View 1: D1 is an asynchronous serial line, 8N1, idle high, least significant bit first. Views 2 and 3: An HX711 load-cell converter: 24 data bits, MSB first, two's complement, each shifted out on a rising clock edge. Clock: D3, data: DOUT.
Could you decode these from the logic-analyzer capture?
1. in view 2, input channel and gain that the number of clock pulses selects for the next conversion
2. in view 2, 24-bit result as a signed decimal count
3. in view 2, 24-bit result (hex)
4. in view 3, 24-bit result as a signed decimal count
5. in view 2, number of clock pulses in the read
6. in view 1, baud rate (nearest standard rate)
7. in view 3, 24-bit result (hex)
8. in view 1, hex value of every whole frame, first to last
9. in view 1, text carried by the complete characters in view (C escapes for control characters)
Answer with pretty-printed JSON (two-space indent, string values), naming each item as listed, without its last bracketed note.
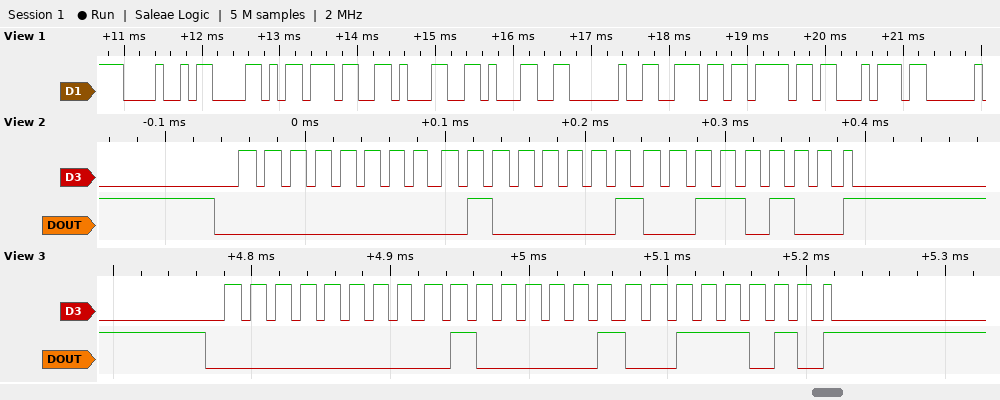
{
  "in view 2, input channel and gain that the number of clock pulses selects for the next conversion": "channel A, gain 128",
  "in view 2, 24-bit result as a signed decimal count": "16692",
  "in view 2, 24-bit result": "0x004134",
  "in view 3, 24-bit result as a signed decimal count": "16698",
  "in view 2, number of clock pulses in the read": "25",
  "in view 1, baud rate": "9600 baud",
  "in view 3, 24-bit result": "0x00413A",
  "in view 1, hex value of every whole frame, first to last": "48 58 37 31 31 20 6E 6F 74",
  "in view 1, text carried by the complete characters in view": "\"HX711 not\""
}
